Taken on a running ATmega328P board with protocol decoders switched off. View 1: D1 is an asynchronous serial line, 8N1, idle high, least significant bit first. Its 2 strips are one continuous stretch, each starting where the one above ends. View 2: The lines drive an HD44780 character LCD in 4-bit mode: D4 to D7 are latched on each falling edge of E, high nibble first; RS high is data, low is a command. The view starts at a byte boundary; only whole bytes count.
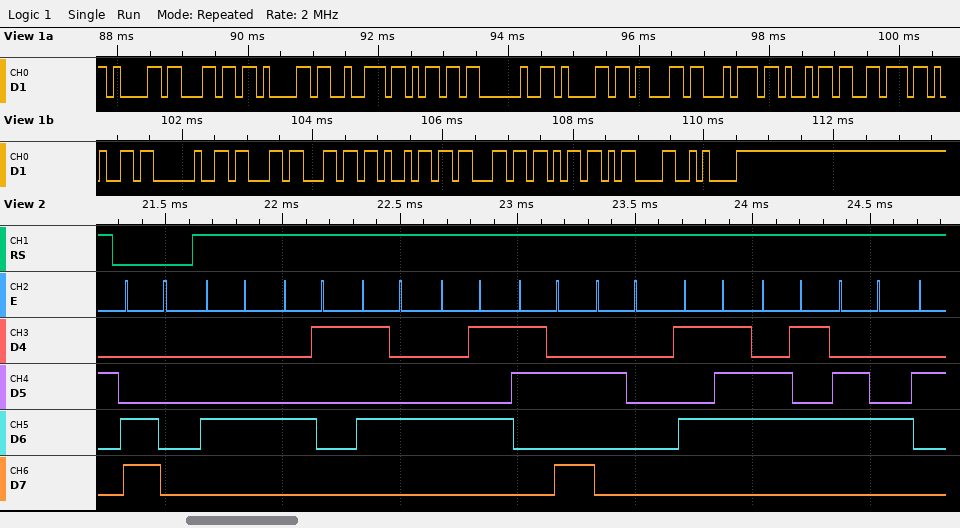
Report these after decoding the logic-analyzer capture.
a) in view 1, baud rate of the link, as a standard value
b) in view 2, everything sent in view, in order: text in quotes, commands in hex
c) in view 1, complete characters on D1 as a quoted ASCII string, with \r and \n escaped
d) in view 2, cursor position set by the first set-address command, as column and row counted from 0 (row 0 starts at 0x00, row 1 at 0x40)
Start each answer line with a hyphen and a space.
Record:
- 9600 baud
- 0xC0 "DATE: Wed"
- "alarm active click\r\n"
- column 0, row 1
